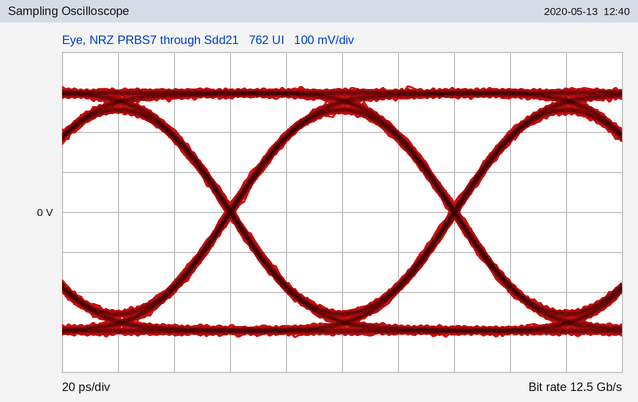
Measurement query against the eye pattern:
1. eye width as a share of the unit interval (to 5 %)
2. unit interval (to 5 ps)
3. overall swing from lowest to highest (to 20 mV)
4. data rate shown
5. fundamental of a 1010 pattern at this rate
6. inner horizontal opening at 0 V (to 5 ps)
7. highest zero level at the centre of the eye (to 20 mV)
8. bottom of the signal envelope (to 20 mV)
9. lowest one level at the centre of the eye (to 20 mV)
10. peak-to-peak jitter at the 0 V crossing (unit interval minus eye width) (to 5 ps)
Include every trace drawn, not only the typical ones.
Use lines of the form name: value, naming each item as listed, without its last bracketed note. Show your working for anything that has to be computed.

eye width as a share of the unit interval: 75 ps / 80 ps ≈ 93.8 %, so 95 % to the nearest 5 %
unit interval: 80 ps
overall swing from lowest to highest: 620 mV
data rate shown: 12.5 Gb/s
fundamental of a 1010 pattern at this rate: 6.25 GHz
inner horizontal opening at 0 V: 75 ps
highest zero level at the centre of the eye: -240 mV
bottom of the signal envelope: -320 mV
lowest one level at the centre of the eye: 240 mV
peak-to-peak jitter at the 0 V crossing (unit interval minus eye width): 5 ps
